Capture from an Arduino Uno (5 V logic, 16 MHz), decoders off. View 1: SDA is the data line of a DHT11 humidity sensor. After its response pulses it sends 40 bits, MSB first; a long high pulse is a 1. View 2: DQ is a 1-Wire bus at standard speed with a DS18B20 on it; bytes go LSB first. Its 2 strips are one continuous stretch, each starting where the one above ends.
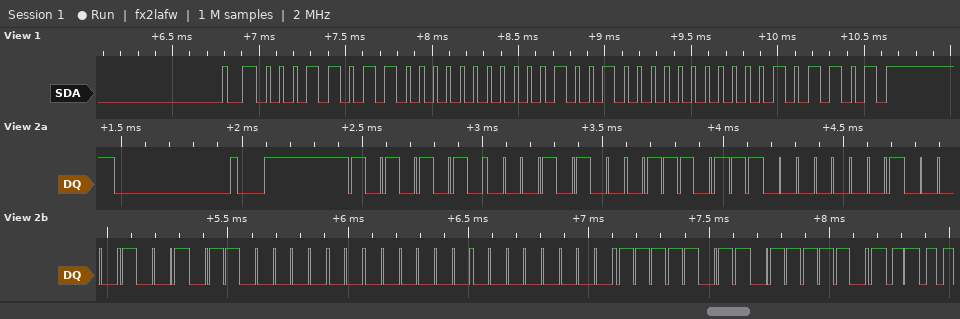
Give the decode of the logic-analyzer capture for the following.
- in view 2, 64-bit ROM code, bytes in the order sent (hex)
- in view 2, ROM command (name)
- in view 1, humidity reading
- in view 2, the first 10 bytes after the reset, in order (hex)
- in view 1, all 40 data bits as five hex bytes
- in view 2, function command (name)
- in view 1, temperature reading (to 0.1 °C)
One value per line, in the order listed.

28 EE 80 90 06 00 00 DF
Match ROM
27 %
55 28 EE 80 90 06 00 00 DF BE
1B 00 12 00 2D
Read Scratchpad
18.0 °C
